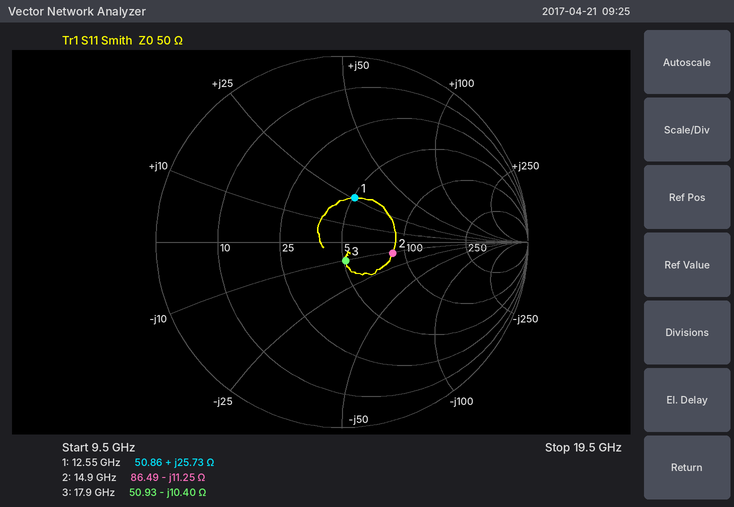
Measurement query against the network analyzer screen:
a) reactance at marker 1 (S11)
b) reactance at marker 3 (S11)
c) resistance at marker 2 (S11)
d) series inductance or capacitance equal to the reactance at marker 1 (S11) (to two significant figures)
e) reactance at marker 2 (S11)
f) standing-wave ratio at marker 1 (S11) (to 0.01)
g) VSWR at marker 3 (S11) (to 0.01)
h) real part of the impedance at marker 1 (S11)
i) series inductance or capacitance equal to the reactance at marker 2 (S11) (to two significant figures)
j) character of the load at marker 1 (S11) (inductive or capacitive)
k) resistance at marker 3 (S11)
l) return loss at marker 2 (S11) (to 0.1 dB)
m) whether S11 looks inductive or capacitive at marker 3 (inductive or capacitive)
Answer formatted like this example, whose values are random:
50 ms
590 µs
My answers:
+25.73 Ω
-10.40 Ω
86.49 Ω
330 pH
-11.25 Ω
1.66
1.23
50.86 Ω
950 fF
inductive
50.93 Ω
11.1 dB
capacitive
